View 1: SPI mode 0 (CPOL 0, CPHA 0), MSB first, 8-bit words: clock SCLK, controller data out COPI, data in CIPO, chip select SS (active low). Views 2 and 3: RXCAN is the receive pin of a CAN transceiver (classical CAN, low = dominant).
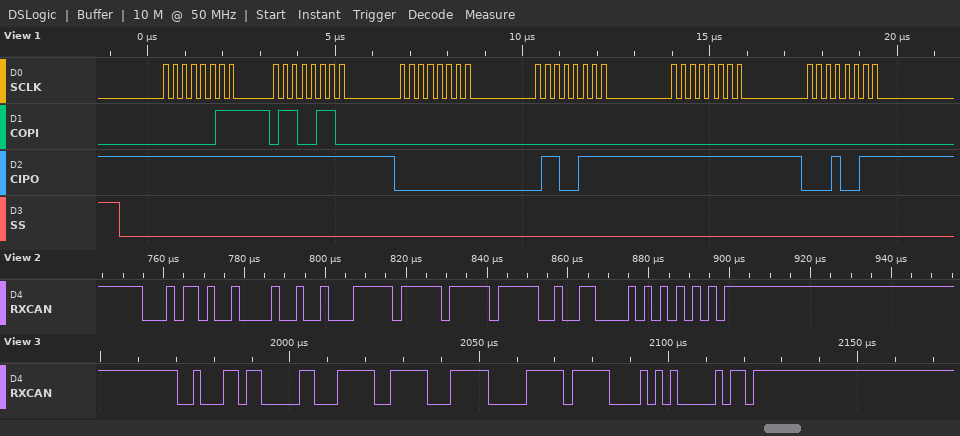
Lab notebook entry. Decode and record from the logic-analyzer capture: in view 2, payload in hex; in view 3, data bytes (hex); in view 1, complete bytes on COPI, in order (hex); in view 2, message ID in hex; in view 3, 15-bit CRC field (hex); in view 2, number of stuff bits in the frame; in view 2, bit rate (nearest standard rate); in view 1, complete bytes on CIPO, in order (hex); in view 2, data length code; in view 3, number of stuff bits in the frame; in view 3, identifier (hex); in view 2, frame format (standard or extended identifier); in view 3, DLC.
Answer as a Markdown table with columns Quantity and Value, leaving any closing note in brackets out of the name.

| Quantity | Value |
|---|---|
| in view 2, payload in hex | 91 FF FF E9 |
| in view 3, data bytes | 7D F3 E1 FF |
| in view 1, complete bytes on COPI, in order | 03 66 00 00 00 00 |
| in view 2, message ID in hex | 0x169 |
| in view 3, 15-bit CRC field | 0x0A81 |
| in view 2, number of stuff bits in the frame | 4 |
| in view 2, bit rate | 500 kbit/s |
| in view 1, complete bytes on CIPO, in order | FF FF 00 67 FF 13 |
| in view 2, data length code | 4 |
| in view 3, number of stuff bits in the frame | 8 |
| in view 3, identifier | 0x236 |
| in view 2, frame format | standard |
| in view 3, DLC | 4 |
